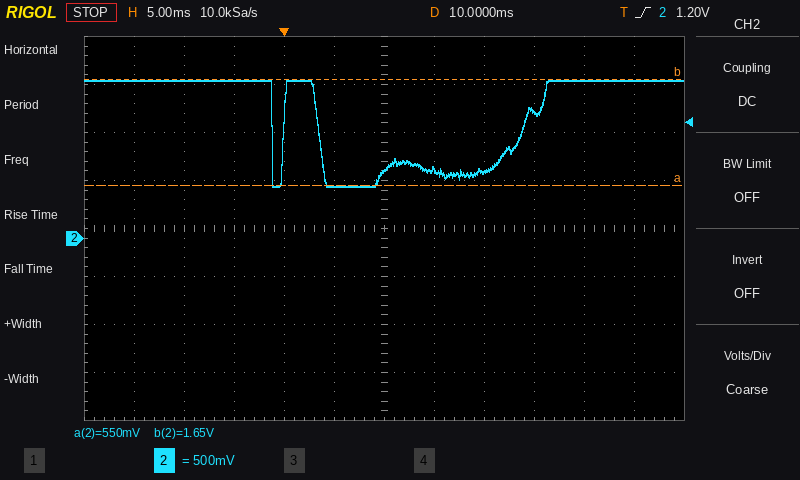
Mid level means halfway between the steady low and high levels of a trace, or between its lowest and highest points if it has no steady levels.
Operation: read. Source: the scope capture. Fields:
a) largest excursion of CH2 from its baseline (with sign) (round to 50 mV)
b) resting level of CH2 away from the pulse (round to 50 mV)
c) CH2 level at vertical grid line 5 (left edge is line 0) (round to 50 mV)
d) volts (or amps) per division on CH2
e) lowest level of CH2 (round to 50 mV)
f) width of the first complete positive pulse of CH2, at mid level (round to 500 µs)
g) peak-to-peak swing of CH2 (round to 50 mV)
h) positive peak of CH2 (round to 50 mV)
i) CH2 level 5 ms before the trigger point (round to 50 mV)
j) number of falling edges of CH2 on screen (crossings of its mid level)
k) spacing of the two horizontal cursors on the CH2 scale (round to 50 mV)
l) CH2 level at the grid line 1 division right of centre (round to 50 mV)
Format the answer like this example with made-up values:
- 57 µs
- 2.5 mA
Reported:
- -1.10 V
- 1.65 V
- 550 mV
- 500 mV
- 550 mV
- 3.5 ms
- 1.10 V
- 1.65 V
- 1.65 V
- 2
- 1.10 V
- 700 mV
